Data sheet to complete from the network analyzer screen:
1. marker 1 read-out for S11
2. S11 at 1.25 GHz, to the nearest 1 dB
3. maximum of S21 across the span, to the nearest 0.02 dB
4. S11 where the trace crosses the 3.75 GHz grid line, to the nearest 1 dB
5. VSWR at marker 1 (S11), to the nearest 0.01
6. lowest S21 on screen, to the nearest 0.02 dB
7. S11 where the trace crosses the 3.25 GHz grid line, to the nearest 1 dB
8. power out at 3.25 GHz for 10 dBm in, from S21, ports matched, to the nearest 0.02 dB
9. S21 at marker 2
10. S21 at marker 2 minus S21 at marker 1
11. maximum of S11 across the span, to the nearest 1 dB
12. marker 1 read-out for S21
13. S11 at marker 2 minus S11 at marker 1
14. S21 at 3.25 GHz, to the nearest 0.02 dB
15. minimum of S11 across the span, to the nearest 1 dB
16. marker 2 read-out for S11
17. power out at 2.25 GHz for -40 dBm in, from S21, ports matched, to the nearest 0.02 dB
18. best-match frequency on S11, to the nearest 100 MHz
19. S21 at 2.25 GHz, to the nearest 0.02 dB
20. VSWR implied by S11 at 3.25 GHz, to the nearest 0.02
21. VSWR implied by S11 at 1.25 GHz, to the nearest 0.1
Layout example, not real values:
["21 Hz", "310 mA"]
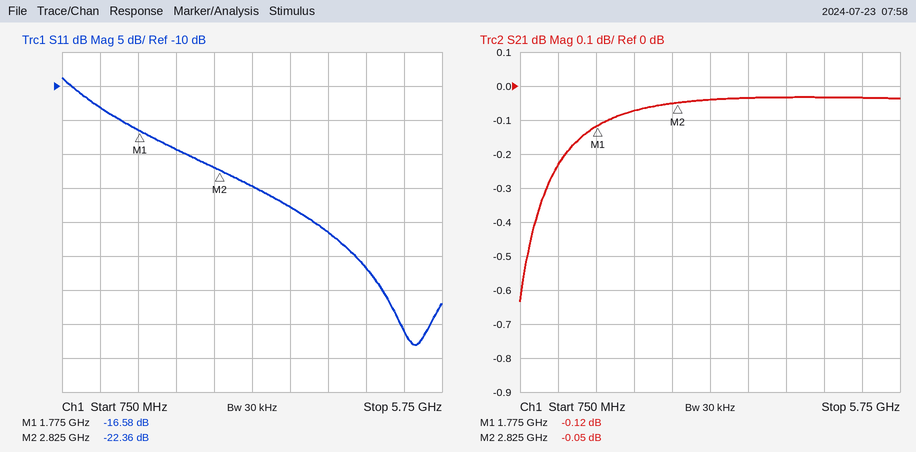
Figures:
["-16.58 dB", "-13 dB", "-0.04 dB", "-28 dB", "1.35", "-0.64 dB", "-25 dB", "9.96 dBm", "-0.05 dB", "0.07 dB", "-9 dB", "-0.12 dB", "-5.78 dB", "-0.04 dB", "-48 dB", "-22.36 dB", "-40.08 dBm", "5.4 GHz", "-0.08 dB", "1.12", "1.6"]
